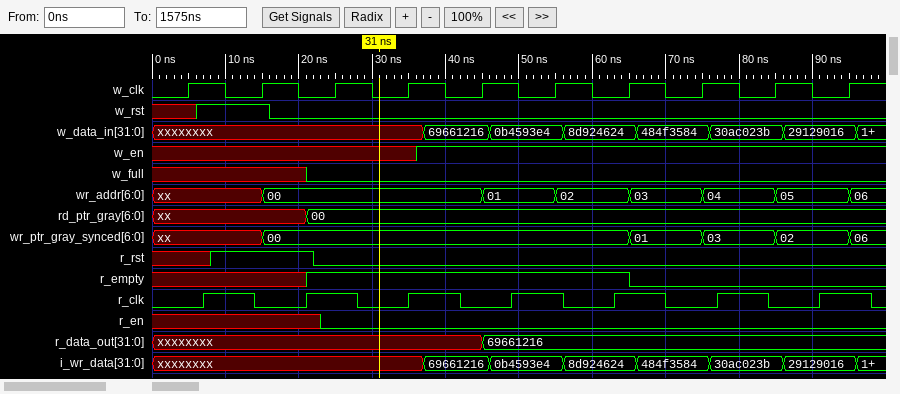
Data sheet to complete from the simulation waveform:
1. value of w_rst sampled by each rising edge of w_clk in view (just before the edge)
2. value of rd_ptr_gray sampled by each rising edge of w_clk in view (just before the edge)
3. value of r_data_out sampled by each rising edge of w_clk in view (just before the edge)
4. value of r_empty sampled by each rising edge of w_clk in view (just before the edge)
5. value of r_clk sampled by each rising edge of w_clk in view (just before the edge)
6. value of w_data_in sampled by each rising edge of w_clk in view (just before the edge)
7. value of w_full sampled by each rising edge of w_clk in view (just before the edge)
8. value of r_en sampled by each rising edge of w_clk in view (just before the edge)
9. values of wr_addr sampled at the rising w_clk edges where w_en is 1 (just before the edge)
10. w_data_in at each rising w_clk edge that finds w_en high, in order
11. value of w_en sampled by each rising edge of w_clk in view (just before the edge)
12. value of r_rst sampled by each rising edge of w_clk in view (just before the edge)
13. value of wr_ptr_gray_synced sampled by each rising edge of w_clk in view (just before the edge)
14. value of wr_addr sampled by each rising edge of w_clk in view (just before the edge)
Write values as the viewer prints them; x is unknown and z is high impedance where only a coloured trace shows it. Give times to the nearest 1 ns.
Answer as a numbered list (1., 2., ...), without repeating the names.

1. x 1 0 0 0 0 0 0 0 0
2. xx, xx, 00, 00, 00, 00, 00, 00, 00, 00
3. xxxxxxxx, xxxxxxxx, xxxxxxxx, xxxxxxxx, xxxxxxxx, 69661216, 69661216, 69661216, 69661216, 69661216
4. x x 1 1 1 1 1 0 0 0
5. 0 0 1 0 0 1 1 0 0 1
6. xxxxxxxx, xxxxxxxx, xxxxxxxx, xxxxxxxx, 69661216, 0b4593e4, 8d924624, 484f3584, 30ac023b, 29129016
7. x x 0 0 0 0 0 0 0 0
8. x x 0 0 0 0 0 0 0 0
9. 00, 01, 02, 03, 04, 05
10. 69661216, 0b4593e4, 8d924624, 484f3584, 30ac023b, 29129016
11. x x x x 1 1 1 1 1 1
12. x 1 0 0 0 0 0 0 0 0
13. xx, xx, 00, 00, 00, 00, 00, 01, 03, 02
14. xx, xx, 00, 00, 00, 01, 02, 03, 04, 05
